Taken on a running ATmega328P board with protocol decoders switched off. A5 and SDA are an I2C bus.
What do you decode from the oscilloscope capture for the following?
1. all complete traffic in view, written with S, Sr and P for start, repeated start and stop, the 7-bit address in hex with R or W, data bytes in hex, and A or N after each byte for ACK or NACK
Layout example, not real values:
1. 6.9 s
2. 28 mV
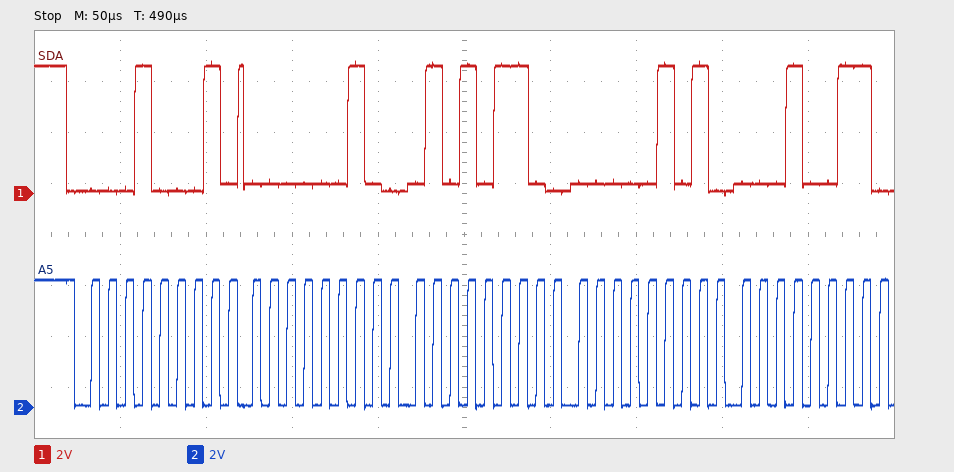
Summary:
1. S 08R A 02 A 56 A 05 A 13 A
